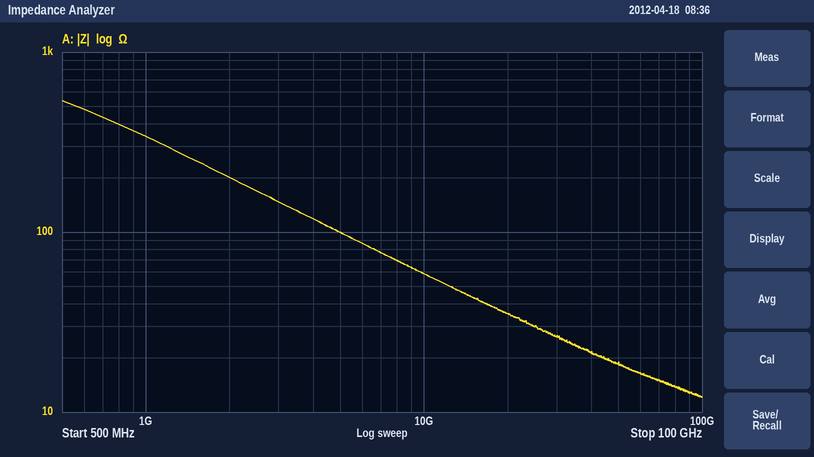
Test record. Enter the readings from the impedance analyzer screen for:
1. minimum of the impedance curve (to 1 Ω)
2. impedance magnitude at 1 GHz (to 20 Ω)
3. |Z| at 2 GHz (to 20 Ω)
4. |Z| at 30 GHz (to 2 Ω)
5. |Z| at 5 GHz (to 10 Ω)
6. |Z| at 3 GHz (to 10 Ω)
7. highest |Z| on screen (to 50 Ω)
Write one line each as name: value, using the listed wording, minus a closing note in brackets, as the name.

minimum of the impedance curve: 12 Ω
impedance magnitude at 1 GHz: 340 Ω
|Z| at 2 GHz: 200 Ω
|Z| at 30 GHz: 26 Ω
|Z| at 5 GHz: 100 Ω
|Z| at 3 GHz: 150 Ω
highest |Z| on screen: 550 Ω
